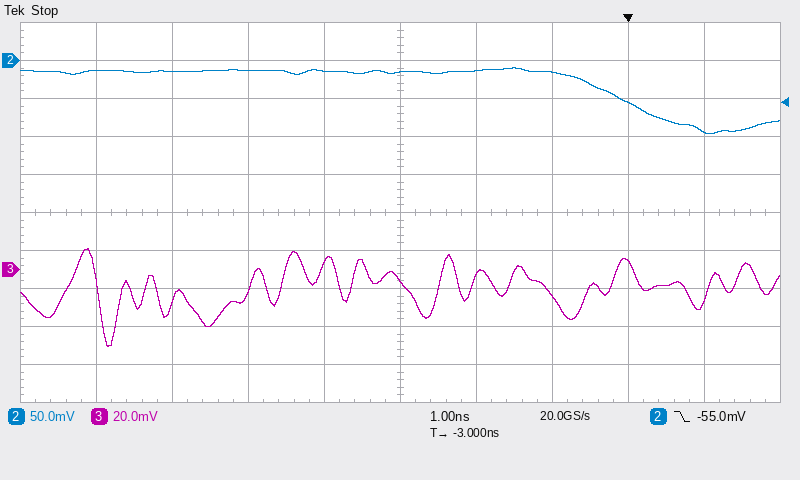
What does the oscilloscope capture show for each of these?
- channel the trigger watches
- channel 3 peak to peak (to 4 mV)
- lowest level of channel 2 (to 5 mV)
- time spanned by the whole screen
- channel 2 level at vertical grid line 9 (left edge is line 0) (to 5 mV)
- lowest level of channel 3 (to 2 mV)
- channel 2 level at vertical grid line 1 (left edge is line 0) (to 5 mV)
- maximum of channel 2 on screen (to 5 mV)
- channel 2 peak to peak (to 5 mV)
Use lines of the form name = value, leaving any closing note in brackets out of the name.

channel the trigger watches = channel 2
channel 3 peak to peak = 52 mV
lowest level of channel 2 = -95 mV
time spanned by the whole screen = 10 ns
channel 2 level at vertical grid line 9 (left edge is line 0) = -95 mV
lowest level of channel 3 = -40 mV
channel 2 level at vertical grid line 1 (left edge is line 0) = -15 mV
maximum of channel 2 on screen = -10 mV
channel 2 peak to peak = 85 mV
